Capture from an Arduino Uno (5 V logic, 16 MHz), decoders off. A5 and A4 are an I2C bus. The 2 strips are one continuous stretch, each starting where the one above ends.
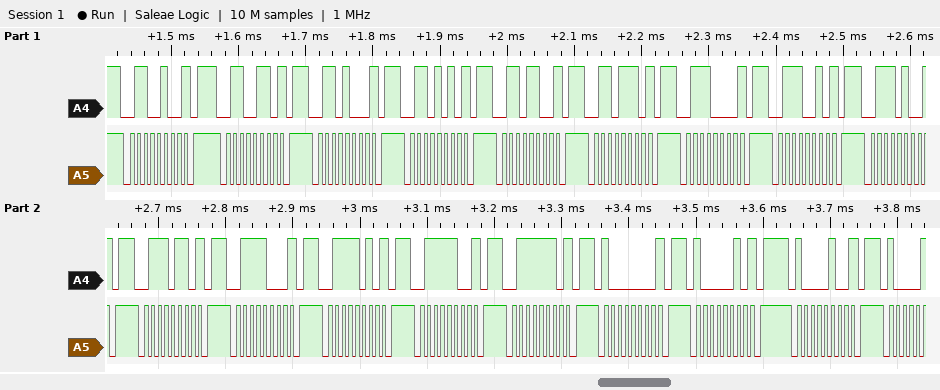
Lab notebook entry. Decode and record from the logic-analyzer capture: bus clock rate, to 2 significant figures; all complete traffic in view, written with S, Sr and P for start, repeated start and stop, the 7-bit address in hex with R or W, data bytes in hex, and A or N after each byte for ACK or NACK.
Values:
100 kHz
S 32W N P S 33W N P S 34W N P S 35W N P S 36W N P S 37W N P S 38W N P S 39W N P S 3AW N P S 3BW N P S 3CW N P S 3DW N P S 3EW N P S 3FW N P S 40W N P S 41W N P S 42W N P
